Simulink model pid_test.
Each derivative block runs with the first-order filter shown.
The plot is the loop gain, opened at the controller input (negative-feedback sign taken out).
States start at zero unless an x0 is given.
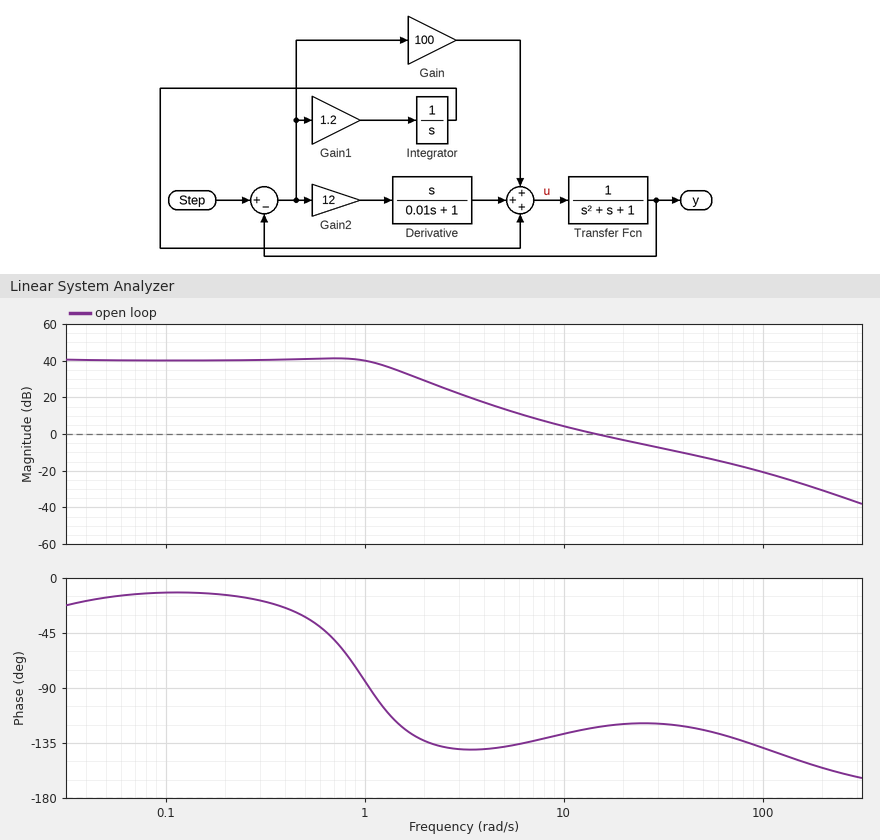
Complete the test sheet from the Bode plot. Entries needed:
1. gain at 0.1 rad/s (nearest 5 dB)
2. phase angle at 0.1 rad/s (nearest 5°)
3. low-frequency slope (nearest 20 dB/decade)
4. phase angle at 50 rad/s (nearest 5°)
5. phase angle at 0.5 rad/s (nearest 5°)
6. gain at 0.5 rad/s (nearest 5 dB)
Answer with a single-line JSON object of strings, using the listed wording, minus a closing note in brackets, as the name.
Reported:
{"gain at 0.1 rad/s": "40 dB", "phase angle at 0.1 rad/s": "-10°", "low-frequency slope": "0 dB/decade", "phase angle at 50 rad/s": "-125°", "phase angle at 0.5 rad/s": "-30°", "gain at 0.5 rad/s": "40 dB"}
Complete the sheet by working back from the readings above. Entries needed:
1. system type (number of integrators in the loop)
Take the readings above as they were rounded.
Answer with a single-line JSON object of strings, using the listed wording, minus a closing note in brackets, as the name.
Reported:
{"system type": "0"}
